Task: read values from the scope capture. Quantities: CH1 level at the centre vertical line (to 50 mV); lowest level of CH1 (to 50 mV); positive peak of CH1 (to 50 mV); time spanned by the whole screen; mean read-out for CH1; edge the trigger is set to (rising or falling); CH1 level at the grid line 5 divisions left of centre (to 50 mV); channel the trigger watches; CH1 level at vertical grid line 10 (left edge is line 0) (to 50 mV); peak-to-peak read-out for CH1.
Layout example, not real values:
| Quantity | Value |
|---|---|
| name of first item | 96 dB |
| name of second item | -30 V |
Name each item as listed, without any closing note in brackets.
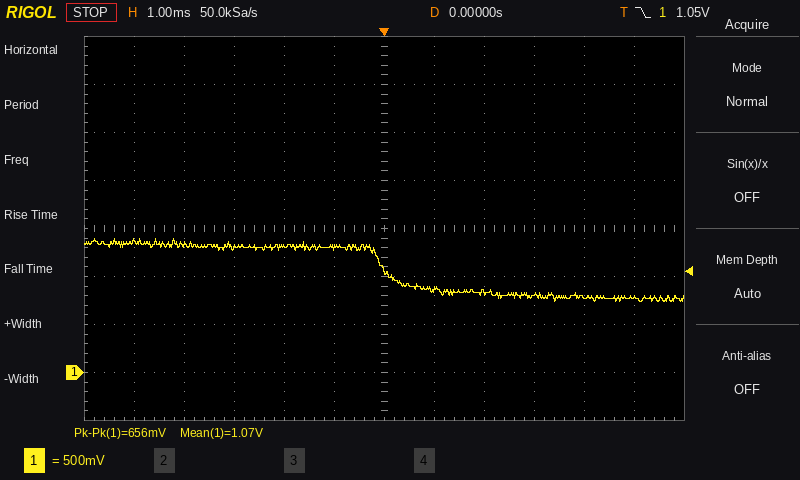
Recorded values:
| Quantity | Value |
|---|---|
| CH1 level at the centre vertical line | 1.05 V |
| lowest level of CH1 | 750 mV |
| positive peak of CH1 | 1.40 V |
| time spanned by the whole screen | 12 ms |
| mean read-out for CH1 | 1.07 V |
| edge the trigger is set to | falling |
| CH1 level at the grid line 5 divisions left of centre | 1.35 V |
| channel the trigger watches | CH1 |
| CH1 level at vertical grid line 10 (left edge is line 0) | 800 mV |
| peak-to-peak read-out for CH1 | 656 mV |
